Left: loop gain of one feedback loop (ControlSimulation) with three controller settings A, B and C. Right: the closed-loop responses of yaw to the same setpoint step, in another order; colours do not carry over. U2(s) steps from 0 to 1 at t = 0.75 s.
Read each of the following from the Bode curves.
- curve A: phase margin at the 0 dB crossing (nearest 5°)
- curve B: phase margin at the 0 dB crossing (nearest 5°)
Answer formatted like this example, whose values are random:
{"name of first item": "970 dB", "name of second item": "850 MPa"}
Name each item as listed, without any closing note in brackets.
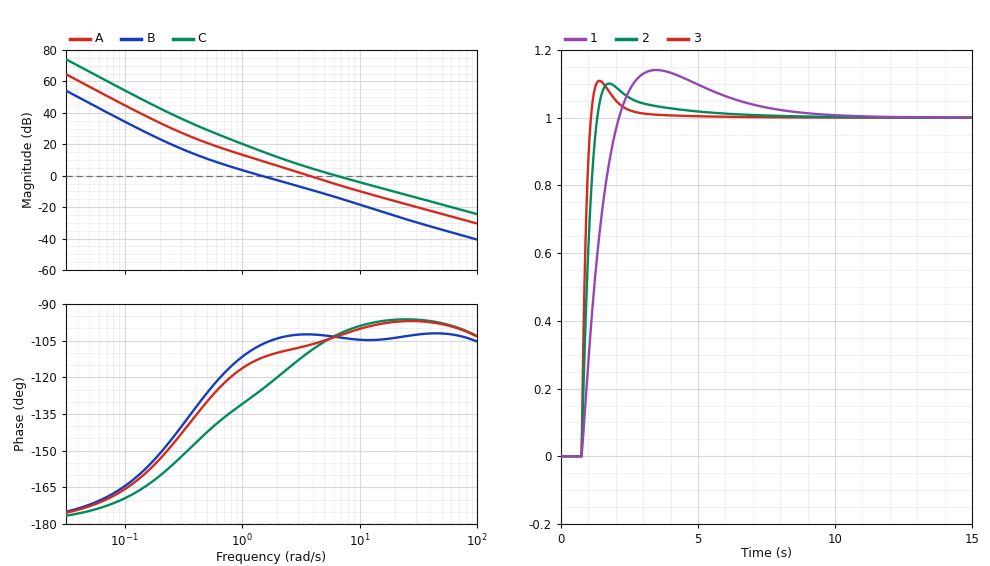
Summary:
{"curve A: phase margin at the 0 dB crossing": "75°", "curve B: phase margin at the 0 dB crossing": "75°"}
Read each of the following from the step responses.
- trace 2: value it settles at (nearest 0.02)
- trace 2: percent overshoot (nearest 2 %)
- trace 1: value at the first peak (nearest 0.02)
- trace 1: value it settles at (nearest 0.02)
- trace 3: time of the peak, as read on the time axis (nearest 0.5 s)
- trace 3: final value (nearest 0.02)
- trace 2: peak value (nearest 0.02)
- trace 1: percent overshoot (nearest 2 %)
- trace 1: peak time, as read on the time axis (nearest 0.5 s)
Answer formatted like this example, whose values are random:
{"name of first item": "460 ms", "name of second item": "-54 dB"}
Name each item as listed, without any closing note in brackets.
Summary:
{"trace 2: value it settles at": "1.00", "trace 2: percent overshoot": "10 %", "trace 1: value at the first peak": "1.14", "trace 1: value it settles at": "1.00", "trace 3: time of the peak, as read on the time axis": "1.5 s", "trace 3: final value": "1.00", "trace 2: peak value": "1.10", "trace 1: percent overshoot": "14 %", "trace 1: peak time, as read on the time axis": "3.5 s"}
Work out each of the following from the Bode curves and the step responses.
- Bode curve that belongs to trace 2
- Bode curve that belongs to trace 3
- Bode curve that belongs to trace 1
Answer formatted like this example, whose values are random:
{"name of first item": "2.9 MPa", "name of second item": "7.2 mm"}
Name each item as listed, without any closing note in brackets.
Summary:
{"Bode curve that belongs to trace 2": "A", "Bode curve that belongs to trace 3": "C", "Bode curve that belongs to trace 1": "B"}
